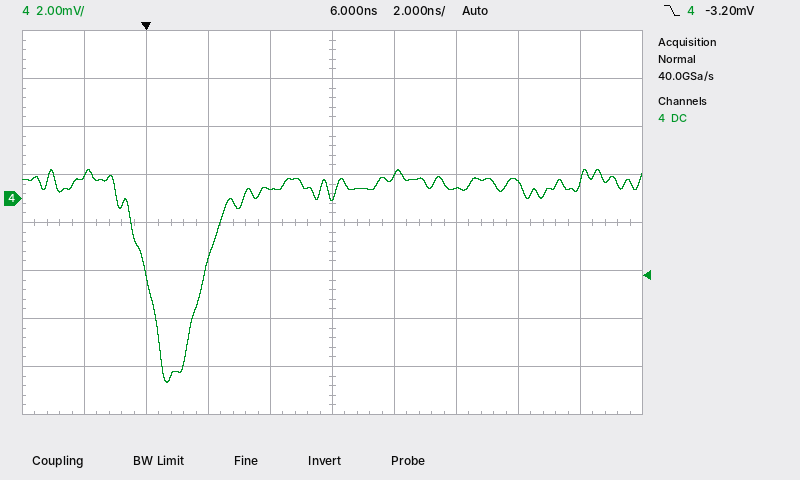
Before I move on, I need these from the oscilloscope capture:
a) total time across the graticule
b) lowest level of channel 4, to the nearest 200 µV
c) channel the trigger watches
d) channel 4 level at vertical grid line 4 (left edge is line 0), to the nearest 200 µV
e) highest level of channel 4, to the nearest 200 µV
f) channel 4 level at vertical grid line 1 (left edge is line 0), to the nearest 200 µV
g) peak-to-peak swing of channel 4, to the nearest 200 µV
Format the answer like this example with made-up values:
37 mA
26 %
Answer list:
20 ns
-7.6 mV
channel 4
400 µV
1.2 mV
1.0 mV
8.8 mV
